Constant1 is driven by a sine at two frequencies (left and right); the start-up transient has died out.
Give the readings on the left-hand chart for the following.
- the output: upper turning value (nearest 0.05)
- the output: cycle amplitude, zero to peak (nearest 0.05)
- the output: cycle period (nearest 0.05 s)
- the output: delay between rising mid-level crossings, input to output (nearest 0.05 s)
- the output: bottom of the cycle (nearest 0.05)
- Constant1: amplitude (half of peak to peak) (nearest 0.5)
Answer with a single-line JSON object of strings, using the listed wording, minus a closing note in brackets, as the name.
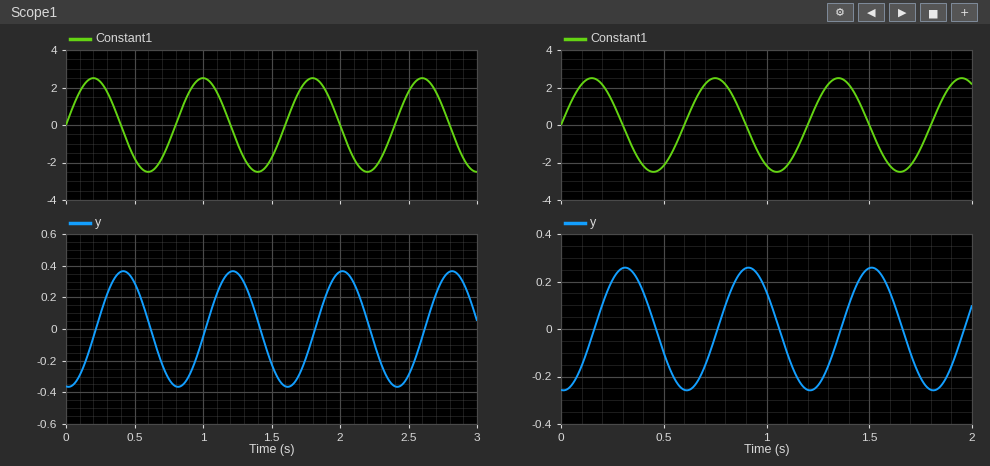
{"the output: upper turning value": "0.35", "the output: cycle amplitude, zero to peak": "0.35", "the output: cycle period": "0.80 s", "the output: delay between rising mid-level crossings, input to output": "0.20 s", "the output: bottom of the cycle": "-0.35", "Constant1: amplitude (half of peak to peak)": "2.5"}
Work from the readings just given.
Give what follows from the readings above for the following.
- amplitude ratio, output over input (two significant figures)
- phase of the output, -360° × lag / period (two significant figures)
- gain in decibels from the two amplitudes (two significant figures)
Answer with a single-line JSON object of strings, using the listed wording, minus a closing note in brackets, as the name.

{"amplitude ratio, output over input": "0.14", "phase of the output, -360° × lag / period": "-90°", "gain in decibels from the two amplitudes": "-17 dB"}
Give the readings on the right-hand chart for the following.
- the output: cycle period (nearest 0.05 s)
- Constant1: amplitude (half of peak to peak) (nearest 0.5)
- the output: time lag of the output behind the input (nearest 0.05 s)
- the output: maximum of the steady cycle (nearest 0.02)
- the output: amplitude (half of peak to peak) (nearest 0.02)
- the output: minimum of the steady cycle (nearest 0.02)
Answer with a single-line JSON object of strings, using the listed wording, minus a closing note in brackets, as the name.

{"the output: cycle period": "0.60 s", "Constant1: amplitude (half of peak to peak)": "2.5", "the output: time lag of the output behind the input": "0.15 s", "the output: maximum of the steady cycle": "0.26", "the output: amplitude (half of peak to peak)": "0.26", "the output: minimum of the steady cycle": "-0.26"}
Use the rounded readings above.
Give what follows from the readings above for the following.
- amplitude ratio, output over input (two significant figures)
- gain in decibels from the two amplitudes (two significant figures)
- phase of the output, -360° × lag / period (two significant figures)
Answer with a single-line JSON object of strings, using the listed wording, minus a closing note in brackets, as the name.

{"amplitude ratio, output over input": "0.10", "gain in decibels from the two amplitudes": "-20 dB", "phase of the output, -360° × lag / period": "-90°"}
